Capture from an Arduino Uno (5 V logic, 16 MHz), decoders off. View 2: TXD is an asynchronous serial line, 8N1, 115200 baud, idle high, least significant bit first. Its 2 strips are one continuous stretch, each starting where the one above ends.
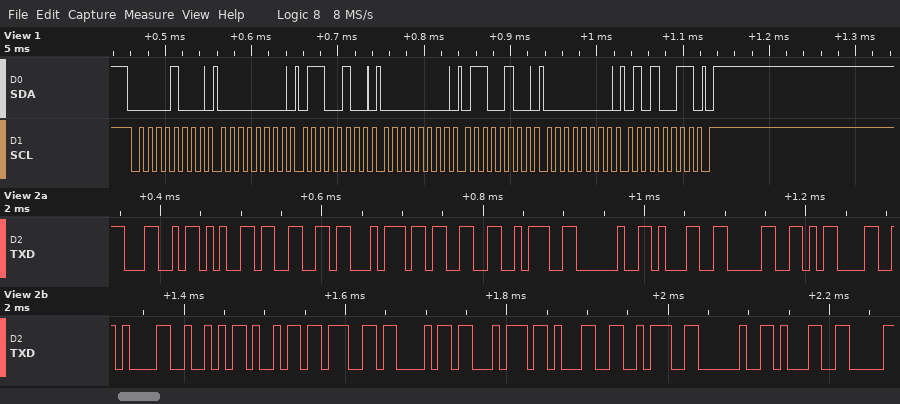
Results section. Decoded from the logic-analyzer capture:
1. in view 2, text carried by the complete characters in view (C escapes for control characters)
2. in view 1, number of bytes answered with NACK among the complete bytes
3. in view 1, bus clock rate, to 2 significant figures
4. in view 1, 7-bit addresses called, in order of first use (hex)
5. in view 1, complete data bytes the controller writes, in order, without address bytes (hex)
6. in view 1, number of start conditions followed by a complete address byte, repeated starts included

"Left3: 10\r\nRight1: 1"
0
100 kHz
0x04
00 64 00 64 00 53
1
